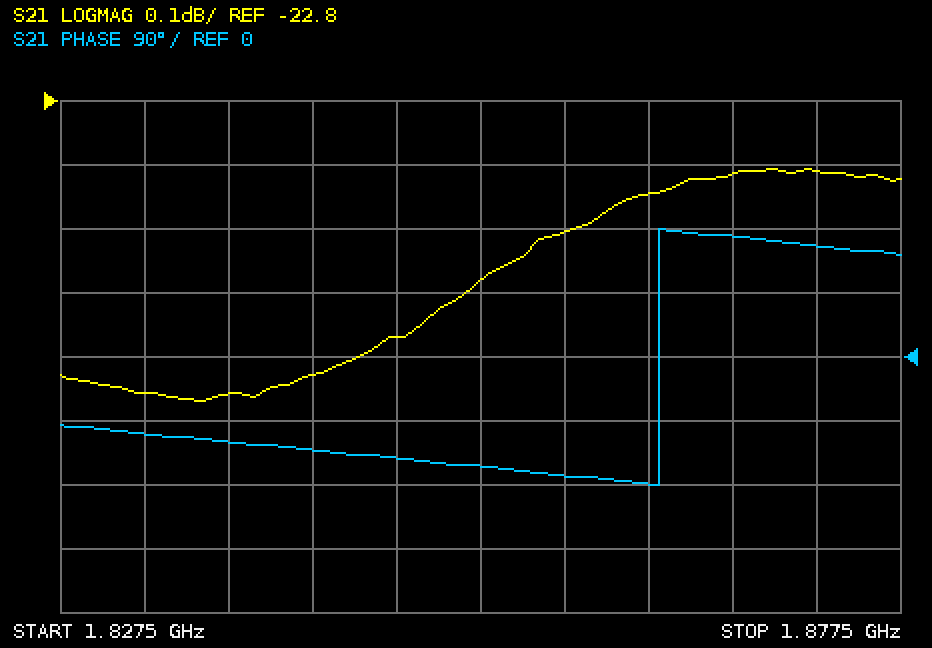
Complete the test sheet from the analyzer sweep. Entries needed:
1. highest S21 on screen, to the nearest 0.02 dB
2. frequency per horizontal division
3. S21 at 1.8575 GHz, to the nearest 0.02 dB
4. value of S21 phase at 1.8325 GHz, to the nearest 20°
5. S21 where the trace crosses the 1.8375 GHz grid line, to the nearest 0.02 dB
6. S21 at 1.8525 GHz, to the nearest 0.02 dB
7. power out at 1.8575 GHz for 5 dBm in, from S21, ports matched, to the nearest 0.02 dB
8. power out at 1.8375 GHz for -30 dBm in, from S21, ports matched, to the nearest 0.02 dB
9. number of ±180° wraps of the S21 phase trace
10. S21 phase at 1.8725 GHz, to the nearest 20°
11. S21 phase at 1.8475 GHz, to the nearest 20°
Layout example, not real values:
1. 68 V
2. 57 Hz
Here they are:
1. -22.90 dB
2. 5 MHz
3. -23.00 dB
4. -100°
5. -23.26 dB
6. -23.08 dB
7. -18.00 dBm
8. -53.26 dBm
9. 1
10. 160°
11. -140°
